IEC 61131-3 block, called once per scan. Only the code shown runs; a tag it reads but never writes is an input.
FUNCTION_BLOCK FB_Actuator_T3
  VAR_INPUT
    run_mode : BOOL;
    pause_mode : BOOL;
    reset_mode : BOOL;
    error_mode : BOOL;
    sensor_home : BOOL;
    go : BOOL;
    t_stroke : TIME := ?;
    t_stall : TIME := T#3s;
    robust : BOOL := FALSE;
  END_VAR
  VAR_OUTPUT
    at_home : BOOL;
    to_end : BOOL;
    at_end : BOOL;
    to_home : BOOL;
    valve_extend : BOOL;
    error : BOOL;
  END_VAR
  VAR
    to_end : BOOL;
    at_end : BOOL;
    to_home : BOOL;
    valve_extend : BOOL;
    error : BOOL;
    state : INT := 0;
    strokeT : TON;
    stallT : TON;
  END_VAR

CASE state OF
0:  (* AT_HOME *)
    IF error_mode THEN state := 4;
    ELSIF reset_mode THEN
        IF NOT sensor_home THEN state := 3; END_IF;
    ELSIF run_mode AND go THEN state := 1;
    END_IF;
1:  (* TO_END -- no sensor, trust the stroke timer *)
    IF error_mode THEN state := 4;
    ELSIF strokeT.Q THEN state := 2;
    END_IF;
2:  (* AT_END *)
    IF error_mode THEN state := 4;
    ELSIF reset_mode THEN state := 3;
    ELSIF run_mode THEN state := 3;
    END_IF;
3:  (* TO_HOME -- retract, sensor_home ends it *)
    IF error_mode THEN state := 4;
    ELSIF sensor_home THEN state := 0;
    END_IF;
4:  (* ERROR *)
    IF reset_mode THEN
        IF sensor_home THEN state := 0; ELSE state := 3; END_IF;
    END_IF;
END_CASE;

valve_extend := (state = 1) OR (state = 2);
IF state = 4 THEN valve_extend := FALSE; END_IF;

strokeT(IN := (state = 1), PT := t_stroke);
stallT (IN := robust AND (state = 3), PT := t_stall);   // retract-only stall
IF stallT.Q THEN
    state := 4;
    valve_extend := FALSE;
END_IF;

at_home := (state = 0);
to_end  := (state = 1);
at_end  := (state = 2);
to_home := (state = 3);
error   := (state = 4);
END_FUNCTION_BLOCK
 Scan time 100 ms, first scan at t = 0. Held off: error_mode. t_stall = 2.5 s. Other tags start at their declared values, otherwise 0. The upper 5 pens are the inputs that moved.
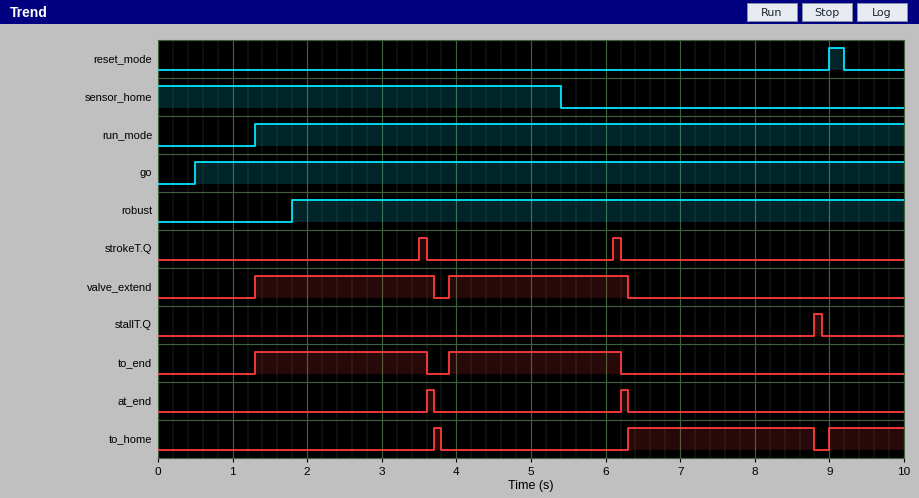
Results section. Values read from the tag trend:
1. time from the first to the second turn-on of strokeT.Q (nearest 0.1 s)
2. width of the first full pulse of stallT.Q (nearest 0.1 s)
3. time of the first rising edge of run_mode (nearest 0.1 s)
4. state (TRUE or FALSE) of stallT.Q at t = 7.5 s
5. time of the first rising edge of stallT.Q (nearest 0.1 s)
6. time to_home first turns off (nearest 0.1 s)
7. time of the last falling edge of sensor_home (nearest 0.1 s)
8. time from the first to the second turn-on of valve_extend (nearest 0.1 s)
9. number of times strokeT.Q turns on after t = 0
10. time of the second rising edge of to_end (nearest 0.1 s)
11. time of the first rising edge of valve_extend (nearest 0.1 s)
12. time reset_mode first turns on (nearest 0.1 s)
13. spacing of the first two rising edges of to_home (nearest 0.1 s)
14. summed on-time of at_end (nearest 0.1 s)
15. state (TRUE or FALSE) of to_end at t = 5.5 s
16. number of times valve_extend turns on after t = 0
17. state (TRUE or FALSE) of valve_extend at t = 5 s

2.6 s
0.1 s
1.3 s
FALSE
8.8 s
3.8 s
5.4 s
2.6 s
2
3.9 s
1.3 s
9.0 s
2.6 s
0.2 s
TRUE
2
TRUE
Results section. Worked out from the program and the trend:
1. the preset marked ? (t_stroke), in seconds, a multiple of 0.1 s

2.2 s
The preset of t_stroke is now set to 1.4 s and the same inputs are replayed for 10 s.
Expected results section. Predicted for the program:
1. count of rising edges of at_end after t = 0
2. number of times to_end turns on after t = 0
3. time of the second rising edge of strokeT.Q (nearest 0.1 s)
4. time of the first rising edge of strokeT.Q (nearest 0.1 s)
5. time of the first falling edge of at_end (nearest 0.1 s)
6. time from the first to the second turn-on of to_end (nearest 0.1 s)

3
3
4.5 s
2.7 s
2.9 s
1.8 s
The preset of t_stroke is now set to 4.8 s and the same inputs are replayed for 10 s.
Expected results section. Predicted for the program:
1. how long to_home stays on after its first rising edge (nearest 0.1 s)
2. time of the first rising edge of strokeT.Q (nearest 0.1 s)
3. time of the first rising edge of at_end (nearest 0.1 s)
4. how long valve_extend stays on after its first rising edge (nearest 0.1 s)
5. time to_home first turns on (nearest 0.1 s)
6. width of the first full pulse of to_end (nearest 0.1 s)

2.5 s
6.1 s
6.2 s
5.0 s
6.3 s
4.9 s
